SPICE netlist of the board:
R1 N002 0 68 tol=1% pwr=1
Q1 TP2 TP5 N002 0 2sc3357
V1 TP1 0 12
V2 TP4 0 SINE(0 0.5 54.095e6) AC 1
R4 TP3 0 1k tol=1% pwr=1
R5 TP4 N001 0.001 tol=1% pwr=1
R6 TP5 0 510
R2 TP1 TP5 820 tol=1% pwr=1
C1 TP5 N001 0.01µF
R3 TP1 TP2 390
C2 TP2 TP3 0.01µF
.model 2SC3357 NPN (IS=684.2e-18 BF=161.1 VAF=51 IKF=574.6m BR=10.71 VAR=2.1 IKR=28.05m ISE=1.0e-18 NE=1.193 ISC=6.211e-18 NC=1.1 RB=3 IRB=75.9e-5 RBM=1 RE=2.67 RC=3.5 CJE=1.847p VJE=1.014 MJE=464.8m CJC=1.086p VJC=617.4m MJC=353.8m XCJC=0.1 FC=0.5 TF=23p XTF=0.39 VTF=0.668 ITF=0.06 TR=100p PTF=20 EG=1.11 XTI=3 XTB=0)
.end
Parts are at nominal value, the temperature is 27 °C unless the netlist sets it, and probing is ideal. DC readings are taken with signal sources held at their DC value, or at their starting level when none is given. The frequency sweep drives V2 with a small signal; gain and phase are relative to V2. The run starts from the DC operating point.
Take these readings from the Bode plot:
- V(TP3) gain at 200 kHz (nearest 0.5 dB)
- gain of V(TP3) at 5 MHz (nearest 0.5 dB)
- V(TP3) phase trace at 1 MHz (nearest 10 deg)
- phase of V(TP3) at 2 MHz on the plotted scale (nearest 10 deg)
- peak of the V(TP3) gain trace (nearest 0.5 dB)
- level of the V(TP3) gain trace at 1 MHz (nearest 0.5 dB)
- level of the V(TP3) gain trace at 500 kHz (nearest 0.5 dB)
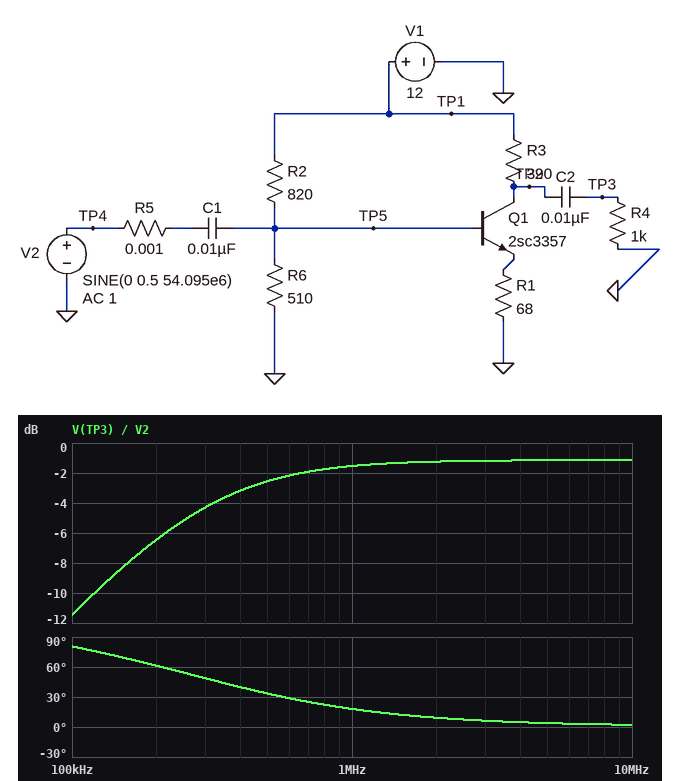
-6.5 dB
-1.0 dB
20 deg
10 deg
-1.0 dB
-1.5 dB
-2.5 dB
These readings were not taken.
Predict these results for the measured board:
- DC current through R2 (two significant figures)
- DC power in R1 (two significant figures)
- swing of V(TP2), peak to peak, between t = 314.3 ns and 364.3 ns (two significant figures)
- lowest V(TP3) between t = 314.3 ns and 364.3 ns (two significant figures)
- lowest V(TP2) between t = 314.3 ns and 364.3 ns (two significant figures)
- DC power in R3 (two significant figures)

11 mA
62 mW
860 mV
-350 mV
1.9 V
240 mW
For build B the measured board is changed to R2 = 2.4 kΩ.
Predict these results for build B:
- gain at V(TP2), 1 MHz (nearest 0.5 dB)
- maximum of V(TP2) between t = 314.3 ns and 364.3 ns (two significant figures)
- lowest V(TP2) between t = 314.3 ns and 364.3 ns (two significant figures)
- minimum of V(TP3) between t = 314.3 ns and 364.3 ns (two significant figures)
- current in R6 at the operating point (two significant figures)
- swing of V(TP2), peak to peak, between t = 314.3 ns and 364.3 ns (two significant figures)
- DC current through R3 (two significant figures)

11.5 dB
7.2 V
3.4 V
-1.9 V
4.0 mA
3.8 V
17 mA
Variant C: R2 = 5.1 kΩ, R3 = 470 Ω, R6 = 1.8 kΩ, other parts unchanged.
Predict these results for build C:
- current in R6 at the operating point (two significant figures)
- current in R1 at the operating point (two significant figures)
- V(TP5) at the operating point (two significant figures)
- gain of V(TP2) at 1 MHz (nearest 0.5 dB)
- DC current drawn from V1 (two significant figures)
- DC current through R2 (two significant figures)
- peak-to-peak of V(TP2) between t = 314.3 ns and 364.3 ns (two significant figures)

1.3 mA
22 mA
2.4 V
-30.5 dB
24 mA
1.9 mA
2.5 V
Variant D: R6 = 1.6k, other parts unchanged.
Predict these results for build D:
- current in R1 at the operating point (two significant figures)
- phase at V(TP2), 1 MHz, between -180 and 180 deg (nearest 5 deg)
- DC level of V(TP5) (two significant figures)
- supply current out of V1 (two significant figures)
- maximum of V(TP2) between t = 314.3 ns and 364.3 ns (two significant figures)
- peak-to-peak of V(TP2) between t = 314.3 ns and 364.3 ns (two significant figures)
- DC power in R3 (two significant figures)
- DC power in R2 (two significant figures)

33 mA
15 deg
3.2 V
35 mA
2.9 V
900 mV
230 mW
94 mW
